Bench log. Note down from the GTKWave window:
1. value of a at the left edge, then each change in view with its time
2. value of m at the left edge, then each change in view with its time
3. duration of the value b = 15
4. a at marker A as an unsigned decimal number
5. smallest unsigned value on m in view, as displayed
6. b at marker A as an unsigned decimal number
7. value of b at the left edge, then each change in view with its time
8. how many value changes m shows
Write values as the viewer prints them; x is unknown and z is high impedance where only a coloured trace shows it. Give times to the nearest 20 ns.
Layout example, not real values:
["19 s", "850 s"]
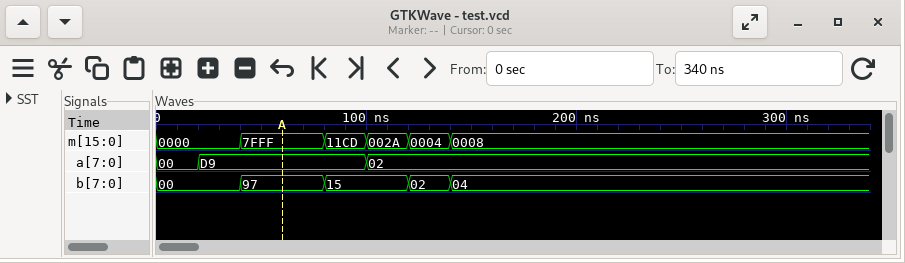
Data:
["00, D9 at 20 ns, 02 at 100 ns", "0000, 7FFF at 40 ns, 11CD at 80 ns, 002A at 100 ns, 0004 at 120 ns, 0008 at 140 ns", "40 ns", "217", "0000", "151", "00, 97 at 40 ns, 15 at 80 ns, 02 at 120 ns, 04 at 140 ns", "5"]
